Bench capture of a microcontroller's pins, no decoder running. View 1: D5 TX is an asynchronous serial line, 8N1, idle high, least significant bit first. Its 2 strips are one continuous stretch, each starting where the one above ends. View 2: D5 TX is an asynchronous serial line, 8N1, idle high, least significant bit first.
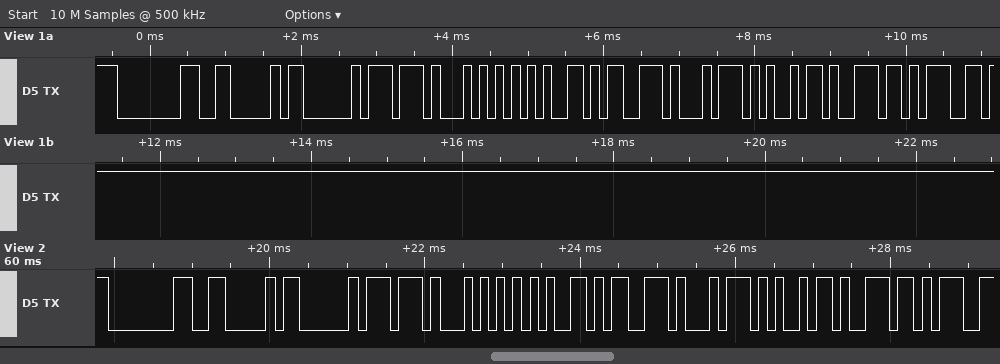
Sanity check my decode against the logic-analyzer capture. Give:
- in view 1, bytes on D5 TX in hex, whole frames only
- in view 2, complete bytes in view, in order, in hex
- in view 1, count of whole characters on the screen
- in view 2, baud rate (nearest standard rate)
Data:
80 06 03 77 54 65 73 74 69 6E 67
0x80 0x06 0x03 0x77 0x54 0x65 0x73 0x74 0x69 0x6E
11
9600 baud
